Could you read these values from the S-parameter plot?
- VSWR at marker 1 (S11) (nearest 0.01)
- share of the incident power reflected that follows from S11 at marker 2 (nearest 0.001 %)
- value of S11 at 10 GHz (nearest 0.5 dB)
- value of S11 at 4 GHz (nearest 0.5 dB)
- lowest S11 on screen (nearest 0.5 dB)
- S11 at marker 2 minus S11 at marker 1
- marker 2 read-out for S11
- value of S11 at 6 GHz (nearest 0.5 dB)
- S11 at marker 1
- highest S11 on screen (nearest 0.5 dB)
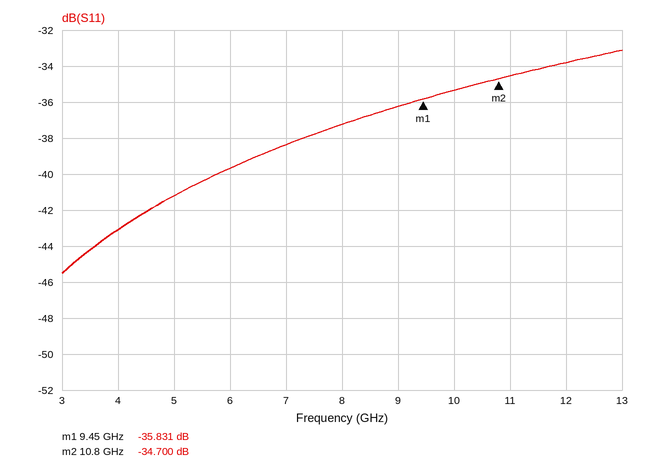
1.03
0.034 %
-35.5 dB
-43.0 dB
-45.5 dB
1.131 dB
-34.700 dB
-39.5 dB
-35.831 dB
-33.0 dB
